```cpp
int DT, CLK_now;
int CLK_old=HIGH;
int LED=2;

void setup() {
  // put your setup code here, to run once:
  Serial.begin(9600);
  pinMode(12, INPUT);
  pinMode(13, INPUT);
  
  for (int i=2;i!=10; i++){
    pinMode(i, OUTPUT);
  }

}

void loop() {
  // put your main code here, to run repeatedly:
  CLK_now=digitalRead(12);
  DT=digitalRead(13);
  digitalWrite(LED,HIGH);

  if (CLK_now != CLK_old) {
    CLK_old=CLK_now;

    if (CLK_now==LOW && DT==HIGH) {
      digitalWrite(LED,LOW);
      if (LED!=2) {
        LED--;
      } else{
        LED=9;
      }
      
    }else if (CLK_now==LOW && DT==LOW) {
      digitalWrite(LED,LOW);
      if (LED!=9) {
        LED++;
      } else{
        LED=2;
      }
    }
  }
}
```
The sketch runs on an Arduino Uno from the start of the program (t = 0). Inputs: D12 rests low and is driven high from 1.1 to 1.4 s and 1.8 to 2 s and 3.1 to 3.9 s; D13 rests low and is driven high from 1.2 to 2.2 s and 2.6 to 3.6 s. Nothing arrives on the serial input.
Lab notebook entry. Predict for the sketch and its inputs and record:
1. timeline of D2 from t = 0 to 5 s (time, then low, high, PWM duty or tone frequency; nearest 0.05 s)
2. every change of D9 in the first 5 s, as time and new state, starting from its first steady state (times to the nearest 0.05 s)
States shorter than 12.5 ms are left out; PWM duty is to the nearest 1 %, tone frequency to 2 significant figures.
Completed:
0 s low; 1.4 s high; 2 s low; 3.9 s high
0 s low; 2 s high; 3.9 s low
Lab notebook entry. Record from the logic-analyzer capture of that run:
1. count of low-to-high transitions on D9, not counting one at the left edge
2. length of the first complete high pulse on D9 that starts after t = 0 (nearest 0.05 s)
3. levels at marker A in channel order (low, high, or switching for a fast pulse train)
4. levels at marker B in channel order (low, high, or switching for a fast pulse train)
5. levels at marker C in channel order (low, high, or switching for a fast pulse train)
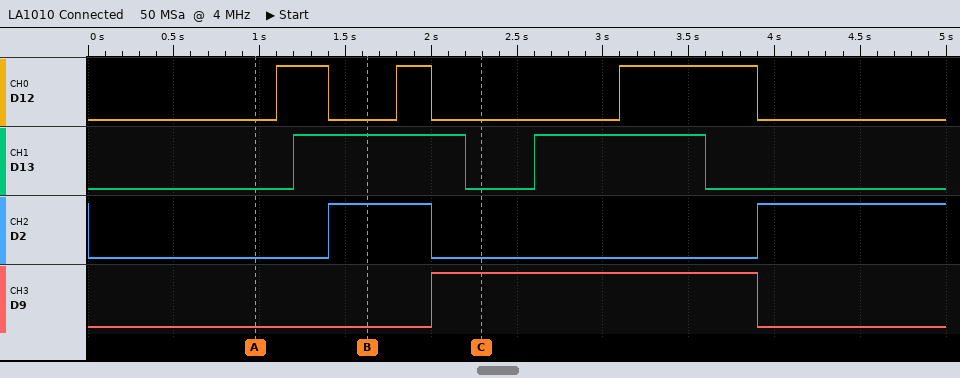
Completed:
1
1.90 s
D12 low, D13 low, D2 low, D9 low
D12 low, D13 high, D2 high, D9 low
D12 low, D13 low, D2 low, D9 high
